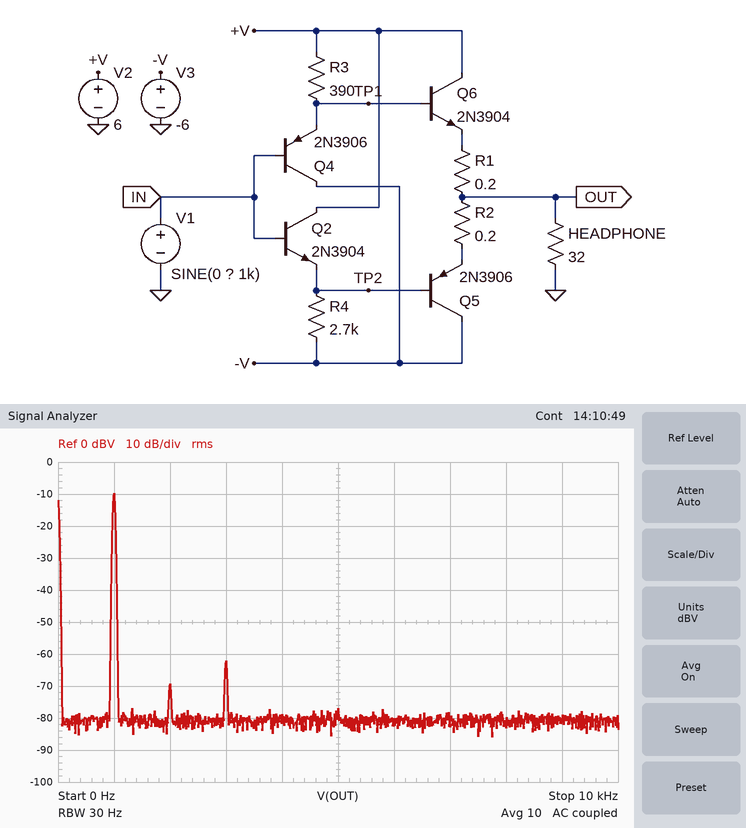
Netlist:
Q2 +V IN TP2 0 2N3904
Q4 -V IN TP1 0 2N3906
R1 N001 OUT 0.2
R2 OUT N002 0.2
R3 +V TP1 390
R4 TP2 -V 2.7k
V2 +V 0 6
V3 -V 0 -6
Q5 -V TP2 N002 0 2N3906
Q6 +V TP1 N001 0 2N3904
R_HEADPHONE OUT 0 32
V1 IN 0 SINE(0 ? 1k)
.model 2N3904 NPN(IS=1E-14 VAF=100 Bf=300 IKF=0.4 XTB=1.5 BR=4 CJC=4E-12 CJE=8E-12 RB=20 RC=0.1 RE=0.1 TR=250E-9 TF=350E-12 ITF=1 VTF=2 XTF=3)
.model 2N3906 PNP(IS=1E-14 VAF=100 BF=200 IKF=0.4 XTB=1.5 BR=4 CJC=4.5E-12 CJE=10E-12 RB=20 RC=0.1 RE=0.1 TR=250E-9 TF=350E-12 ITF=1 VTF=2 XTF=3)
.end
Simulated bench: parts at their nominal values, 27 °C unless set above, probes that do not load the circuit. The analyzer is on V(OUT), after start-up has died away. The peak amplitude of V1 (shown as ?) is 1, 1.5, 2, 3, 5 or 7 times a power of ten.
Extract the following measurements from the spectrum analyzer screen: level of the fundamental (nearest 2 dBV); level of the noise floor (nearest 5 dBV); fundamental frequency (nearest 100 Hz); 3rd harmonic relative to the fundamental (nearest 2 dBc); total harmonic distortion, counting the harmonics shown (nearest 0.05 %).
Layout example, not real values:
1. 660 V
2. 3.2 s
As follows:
1. -10 dBV
2. -80 dBV
3. 1.0 kHz
4. -52 dBc
5. 0.25 %
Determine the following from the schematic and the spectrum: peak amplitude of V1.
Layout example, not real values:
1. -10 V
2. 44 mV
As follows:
1. 500 mV
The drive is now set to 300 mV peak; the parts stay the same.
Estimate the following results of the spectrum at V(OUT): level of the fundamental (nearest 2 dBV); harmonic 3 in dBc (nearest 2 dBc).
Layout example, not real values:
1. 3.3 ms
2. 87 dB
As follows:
1. -14 dBV
2. -58 dBc
